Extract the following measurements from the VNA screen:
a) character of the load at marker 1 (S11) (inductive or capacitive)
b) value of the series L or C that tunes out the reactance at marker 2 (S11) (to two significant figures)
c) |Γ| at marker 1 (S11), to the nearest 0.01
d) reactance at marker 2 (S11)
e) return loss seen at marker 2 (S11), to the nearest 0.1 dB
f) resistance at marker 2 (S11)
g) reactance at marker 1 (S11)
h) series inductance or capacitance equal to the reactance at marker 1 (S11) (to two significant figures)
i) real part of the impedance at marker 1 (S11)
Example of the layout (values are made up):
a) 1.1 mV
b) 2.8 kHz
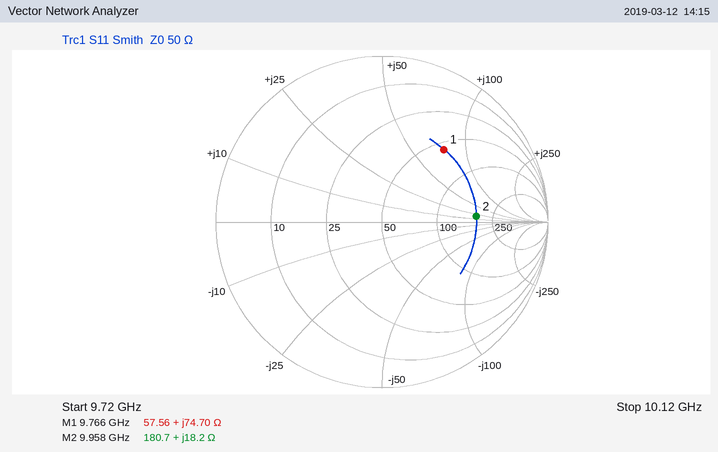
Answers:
a) inductive
b) 880 fF
c) 0.57
d) +18.2 Ω
e) 4.9 dB
f) 180.7 Ω
g) +74.70 Ω
h) 1.2 nH
i) 57.56 Ω
